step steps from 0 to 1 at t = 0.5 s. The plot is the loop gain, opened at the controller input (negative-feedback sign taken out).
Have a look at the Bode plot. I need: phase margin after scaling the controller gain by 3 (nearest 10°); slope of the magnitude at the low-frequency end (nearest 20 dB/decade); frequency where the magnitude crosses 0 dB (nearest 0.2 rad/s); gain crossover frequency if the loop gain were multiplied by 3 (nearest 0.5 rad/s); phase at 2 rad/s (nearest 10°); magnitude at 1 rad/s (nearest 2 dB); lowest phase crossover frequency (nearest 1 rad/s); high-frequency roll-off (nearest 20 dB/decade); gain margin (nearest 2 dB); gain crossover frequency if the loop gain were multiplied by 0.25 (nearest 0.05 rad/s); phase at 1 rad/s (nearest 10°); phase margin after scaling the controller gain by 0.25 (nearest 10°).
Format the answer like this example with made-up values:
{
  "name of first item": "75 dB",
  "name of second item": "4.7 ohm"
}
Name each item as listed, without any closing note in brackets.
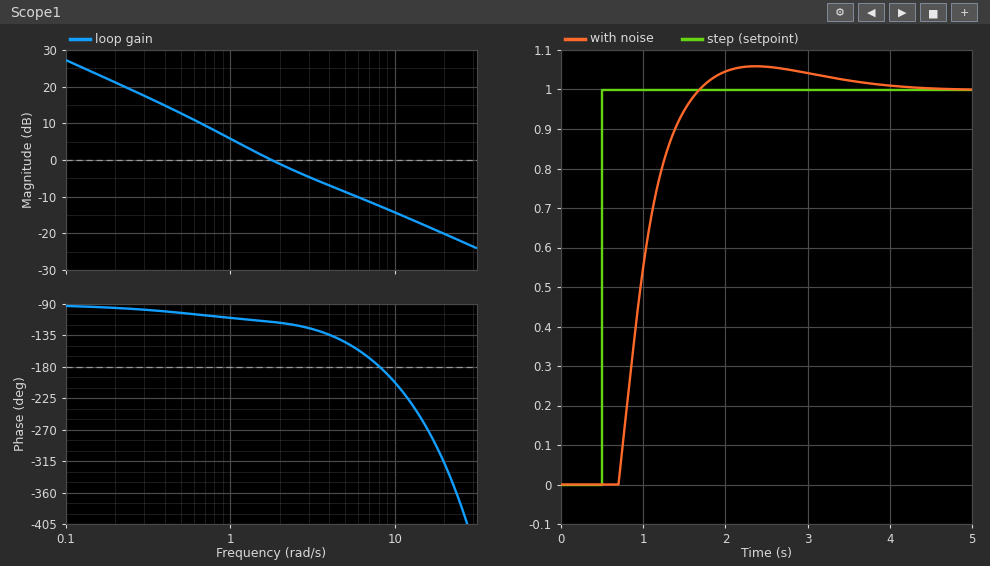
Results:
{
  "phase margin after scaling the controller gain by 3": "30°",
  "slope of the magnitude at the low-frequency end": "-20 dB/decade",
  "frequency where the magnitude crosses 0 dB": "1.8 rad/s",
  "gain crossover frequency if the loop gain were multiplied by 3": "5.5 rad/s",
  "phase at 2 rad/s": "-120°",
  "magnitude at 1 rad/s": "6 dB",
  "lowest phase crossover frequency": "8 rad/s",
  "high-frequency roll-off": "-20 dB/decade",
  "gain margin": "12 dB",
  "gain crossover frequency if the loop gain were multiplied by 0.25": "0.55 rad/s",
  "phase at 1 rad/s": "-110°",
  "phase margin after scaling the controller gain by 0.25": "80°"
}
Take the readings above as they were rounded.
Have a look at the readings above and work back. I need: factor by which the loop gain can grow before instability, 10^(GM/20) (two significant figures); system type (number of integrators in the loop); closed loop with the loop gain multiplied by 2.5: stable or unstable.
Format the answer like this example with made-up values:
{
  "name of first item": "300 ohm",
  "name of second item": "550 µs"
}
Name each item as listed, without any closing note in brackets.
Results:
{
  "factor by which the loop gain can grow before instability, 10^(GM/20)": "4.0",
  "system type": "1",
  "closed loop with the loop gain multiplied by 2.5: stable or unstable": "stable"
}
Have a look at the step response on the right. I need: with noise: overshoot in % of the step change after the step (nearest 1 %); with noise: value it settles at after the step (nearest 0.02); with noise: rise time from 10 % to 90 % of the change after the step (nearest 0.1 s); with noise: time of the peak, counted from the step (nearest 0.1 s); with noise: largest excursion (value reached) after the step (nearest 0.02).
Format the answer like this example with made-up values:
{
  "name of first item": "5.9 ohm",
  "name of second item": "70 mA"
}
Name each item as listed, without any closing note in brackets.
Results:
{
  "with noise: overshoot in % of the step change after the step": "6 %",
  "with noise: value it settles at after the step": "1.00",
  "with noise: rise time from 10 % to 90 % of the change after the step": "0.6 s",
  "with noise: time of the peak, counted from the step": "1.9 s",
  "with noise: largest excursion (value reached) after the step": "1.06"
}
